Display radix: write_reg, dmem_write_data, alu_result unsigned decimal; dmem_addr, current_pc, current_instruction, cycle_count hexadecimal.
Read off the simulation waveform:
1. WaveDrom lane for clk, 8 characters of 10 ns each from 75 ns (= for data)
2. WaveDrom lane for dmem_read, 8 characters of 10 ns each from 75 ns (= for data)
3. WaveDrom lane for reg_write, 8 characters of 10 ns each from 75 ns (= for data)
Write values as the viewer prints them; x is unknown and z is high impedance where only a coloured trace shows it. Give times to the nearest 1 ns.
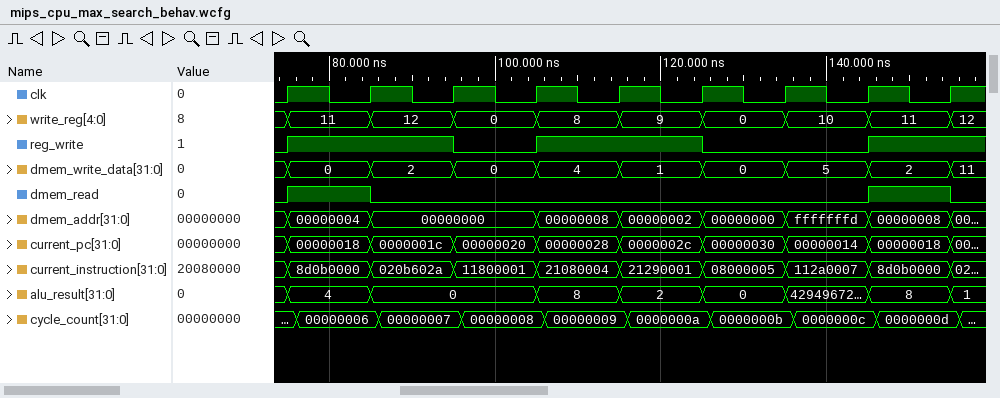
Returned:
{name: 'clk', wave: 'p.......'}
{name: 'dmem_read', wave: '10.....1'}
{name: 'reg_write', wave: '1.01.0.1'}
